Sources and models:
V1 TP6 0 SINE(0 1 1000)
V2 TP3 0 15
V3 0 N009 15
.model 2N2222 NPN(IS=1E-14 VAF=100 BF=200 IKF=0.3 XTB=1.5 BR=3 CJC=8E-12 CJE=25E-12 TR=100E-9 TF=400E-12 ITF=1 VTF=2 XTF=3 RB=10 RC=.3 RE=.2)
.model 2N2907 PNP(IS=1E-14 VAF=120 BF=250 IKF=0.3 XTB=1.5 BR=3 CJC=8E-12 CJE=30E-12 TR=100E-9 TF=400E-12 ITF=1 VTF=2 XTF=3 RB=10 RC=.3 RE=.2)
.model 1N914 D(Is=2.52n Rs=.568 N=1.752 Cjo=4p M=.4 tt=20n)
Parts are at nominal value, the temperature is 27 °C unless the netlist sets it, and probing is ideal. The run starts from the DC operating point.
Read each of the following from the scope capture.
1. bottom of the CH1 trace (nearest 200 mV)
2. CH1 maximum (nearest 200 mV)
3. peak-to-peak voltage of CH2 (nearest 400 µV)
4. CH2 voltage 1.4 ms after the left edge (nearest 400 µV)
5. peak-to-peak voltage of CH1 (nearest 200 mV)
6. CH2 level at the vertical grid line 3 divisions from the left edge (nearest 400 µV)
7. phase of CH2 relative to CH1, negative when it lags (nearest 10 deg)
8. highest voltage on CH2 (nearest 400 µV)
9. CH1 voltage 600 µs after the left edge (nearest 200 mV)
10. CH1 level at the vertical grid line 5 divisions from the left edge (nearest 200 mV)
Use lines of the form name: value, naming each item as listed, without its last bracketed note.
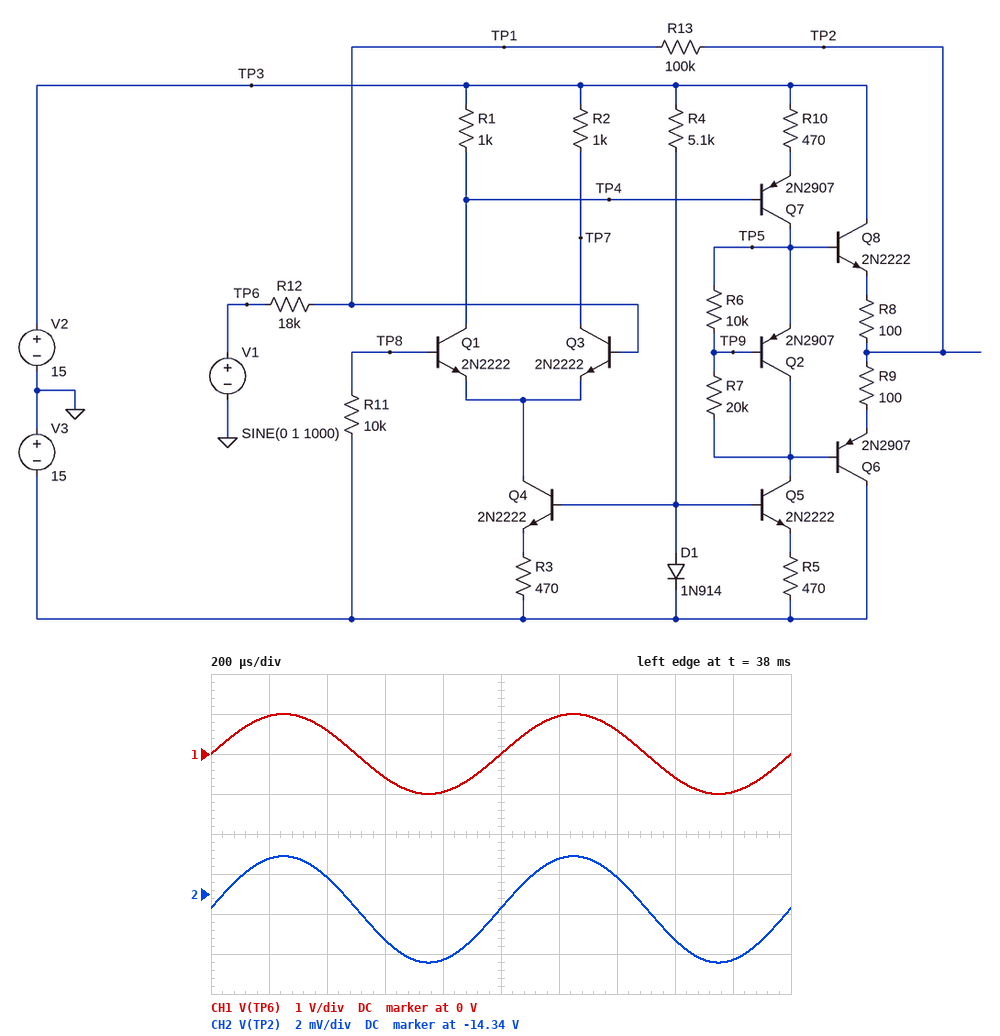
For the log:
bottom of the CH1 trace: -1.0 V
CH1 maximum: 1.0 V
peak-to-peak voltage of CH2: 5.2 mV
CH2 voltage 1.4 ms after the left edge: -14.3392 V
peak-to-peak voltage of CH1: 2.0 V
CH2 level at the vertical grid line 3 divisions from the left edge: -14.3424 V
phase of CH2 relative to CH1, negative when it lags: 0 deg
highest voltage on CH2: -14.3380 V
CH1 voltage 600 µs after the left edge: -600 mV
CH1 level at the vertical grid line 5 divisions from the left edge: 0 V
